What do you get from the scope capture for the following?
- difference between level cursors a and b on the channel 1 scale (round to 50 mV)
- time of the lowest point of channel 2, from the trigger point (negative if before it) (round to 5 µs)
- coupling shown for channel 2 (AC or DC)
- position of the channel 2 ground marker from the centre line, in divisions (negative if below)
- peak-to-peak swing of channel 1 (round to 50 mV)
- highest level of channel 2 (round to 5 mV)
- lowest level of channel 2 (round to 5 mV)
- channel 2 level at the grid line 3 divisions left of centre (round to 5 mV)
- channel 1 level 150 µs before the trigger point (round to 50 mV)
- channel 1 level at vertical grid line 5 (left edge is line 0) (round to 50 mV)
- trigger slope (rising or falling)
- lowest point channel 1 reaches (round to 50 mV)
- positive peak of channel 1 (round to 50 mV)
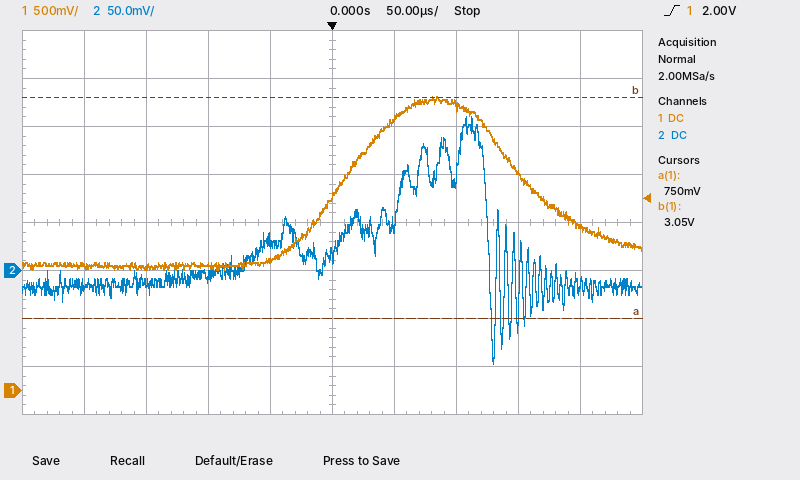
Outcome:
2.30 V
+130 µs
DC
-1.0 div
1.80 V
160 mV
-95 mV
-15 mV
1.30 V
2.00 V
rising
1.25 V
3.05 V
